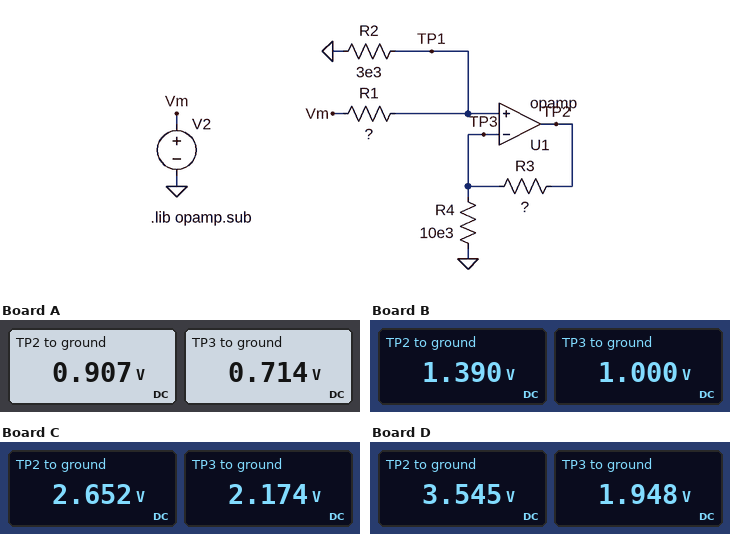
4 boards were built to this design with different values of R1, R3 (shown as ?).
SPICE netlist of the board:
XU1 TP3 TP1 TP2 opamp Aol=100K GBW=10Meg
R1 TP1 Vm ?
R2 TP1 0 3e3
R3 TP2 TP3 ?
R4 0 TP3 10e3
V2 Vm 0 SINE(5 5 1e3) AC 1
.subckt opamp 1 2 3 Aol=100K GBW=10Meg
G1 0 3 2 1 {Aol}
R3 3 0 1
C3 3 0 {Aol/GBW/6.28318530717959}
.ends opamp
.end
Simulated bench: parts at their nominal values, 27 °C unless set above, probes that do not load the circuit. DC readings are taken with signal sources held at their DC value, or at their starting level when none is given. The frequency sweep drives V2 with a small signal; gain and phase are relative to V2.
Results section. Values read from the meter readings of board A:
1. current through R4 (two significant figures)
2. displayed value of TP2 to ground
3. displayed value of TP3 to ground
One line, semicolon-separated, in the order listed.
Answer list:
71 µA; 0.907 V; 0.714 V
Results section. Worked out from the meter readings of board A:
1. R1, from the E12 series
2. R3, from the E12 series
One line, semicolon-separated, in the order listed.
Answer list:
18 kΩ; 2.7 kΩ
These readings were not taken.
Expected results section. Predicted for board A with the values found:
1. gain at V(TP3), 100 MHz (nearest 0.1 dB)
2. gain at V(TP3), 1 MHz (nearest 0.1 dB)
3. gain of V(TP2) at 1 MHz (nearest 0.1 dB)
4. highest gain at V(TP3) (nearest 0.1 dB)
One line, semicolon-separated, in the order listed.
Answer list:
-39.0 dB; -17.0 dB; -14.9 dB; -16.9 dB
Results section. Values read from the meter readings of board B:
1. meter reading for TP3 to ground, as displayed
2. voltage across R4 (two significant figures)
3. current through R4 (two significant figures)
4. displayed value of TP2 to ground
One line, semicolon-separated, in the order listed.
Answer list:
1.000 V; 1.0 V; 100 µA; 1.390 V
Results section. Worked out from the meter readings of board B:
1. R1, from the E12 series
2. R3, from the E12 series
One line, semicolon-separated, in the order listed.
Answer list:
12 kΩ; 3.9 kΩ
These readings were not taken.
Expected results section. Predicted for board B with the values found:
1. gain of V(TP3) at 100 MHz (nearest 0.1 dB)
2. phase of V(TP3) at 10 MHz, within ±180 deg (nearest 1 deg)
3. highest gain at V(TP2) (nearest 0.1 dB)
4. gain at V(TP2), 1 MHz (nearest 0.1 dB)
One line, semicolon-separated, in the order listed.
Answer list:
-36.9 dB; -54 deg; -11.1 dB; -11.2 dB
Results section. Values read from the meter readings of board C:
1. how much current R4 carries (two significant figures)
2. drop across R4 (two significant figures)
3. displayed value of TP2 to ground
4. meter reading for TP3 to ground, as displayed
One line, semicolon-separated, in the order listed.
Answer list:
220 µA; 2.2 V; 2.652 V; 2.174 V
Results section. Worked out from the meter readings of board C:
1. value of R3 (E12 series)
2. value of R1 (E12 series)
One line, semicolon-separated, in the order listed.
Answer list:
2.2 kΩ; 3.9 kΩ
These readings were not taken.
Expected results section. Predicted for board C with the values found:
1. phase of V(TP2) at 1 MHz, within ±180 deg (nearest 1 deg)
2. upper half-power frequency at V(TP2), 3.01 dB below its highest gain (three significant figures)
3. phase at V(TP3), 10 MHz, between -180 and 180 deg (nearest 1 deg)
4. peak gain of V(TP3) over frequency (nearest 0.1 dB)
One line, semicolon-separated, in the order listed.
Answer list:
-7 deg; 8.20 MHz; -51 deg; -7.2 dB
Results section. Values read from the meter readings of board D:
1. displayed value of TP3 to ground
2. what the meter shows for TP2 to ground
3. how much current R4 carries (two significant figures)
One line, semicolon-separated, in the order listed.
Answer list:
1.948 V; 3.545 V; 190 µA
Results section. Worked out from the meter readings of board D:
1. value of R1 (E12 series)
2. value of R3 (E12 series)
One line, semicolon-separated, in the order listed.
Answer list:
4.7 kΩ; 8.2 kΩ
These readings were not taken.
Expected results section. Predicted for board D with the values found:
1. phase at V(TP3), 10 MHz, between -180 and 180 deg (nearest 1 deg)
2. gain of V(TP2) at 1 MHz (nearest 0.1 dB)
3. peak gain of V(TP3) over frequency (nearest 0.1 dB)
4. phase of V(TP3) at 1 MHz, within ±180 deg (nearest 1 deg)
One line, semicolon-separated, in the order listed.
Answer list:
-61 deg; -3.1 dB; -8.2 dB; -10 deg
